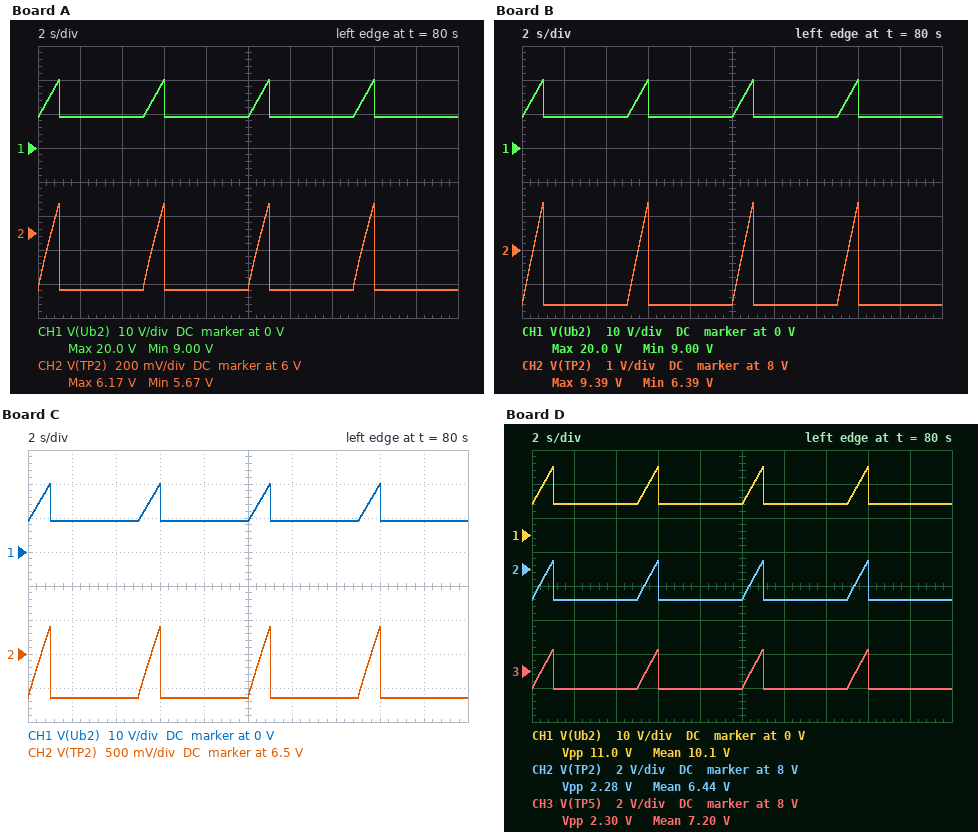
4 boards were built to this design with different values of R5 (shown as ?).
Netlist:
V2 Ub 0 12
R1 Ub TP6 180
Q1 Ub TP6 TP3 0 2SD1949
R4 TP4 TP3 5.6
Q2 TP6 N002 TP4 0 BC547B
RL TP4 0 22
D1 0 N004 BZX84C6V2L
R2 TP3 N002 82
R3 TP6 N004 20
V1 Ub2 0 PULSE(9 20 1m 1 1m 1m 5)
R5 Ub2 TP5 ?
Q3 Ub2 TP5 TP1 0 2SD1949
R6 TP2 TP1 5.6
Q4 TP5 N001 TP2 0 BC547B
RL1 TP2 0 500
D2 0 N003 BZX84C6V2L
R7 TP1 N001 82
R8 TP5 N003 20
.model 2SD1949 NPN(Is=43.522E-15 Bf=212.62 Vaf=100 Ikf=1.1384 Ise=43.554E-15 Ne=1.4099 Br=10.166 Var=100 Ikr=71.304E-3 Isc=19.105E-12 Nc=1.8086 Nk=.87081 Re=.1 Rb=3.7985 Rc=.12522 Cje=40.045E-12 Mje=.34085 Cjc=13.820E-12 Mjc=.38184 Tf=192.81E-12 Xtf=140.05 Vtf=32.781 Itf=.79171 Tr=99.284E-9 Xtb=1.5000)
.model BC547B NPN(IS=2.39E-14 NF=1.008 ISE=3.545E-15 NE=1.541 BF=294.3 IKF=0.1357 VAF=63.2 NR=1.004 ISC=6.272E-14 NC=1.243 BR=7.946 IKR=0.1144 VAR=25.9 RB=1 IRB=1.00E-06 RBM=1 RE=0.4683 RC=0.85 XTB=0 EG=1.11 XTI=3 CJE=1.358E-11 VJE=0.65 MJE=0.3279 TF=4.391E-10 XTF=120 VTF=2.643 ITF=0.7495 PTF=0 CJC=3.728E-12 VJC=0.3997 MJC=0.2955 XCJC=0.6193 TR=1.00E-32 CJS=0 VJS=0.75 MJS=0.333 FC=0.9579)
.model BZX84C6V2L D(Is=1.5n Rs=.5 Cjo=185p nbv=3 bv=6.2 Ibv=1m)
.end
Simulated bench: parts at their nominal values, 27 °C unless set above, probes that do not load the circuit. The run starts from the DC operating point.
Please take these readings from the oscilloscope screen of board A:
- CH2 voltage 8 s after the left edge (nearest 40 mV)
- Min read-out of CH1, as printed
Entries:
5.68 V
9.00 V
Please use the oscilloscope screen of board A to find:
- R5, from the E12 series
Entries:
560 Ω
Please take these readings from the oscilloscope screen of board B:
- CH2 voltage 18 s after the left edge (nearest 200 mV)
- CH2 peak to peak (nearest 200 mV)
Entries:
6.4 V
3.0 V
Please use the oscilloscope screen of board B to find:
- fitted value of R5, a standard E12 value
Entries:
56 Ω
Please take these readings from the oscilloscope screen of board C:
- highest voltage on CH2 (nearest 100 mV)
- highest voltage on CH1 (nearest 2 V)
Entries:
6.9 V
20 V
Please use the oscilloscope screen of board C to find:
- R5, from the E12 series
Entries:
220 Ω
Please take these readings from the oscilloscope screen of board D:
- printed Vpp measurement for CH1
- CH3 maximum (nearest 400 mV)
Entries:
11.0 V
9.2 V
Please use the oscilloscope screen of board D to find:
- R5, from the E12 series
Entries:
82 Ω
